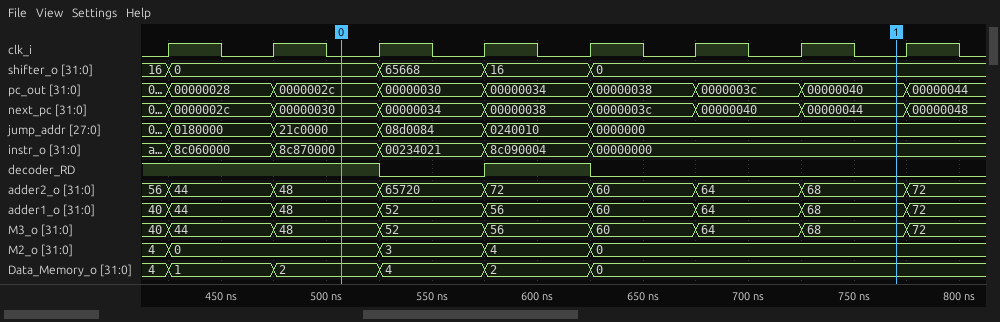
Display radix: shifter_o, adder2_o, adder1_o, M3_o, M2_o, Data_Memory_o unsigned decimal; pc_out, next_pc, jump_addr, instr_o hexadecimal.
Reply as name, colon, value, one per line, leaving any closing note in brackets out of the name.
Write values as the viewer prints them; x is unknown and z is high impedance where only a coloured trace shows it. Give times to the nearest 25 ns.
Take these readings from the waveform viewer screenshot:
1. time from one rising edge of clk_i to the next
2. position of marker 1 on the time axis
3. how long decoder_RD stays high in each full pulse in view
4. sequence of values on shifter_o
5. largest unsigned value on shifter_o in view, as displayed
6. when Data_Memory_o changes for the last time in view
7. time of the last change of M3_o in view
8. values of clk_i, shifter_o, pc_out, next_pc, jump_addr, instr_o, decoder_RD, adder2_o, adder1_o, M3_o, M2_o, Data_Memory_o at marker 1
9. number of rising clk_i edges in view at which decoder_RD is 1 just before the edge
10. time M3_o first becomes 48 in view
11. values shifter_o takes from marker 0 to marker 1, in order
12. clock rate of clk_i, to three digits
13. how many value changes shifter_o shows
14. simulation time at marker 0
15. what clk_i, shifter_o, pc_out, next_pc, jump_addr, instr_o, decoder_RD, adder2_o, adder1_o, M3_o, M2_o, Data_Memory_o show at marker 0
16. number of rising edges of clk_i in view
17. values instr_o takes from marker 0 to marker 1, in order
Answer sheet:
time from one rising edge of clk_i to the next: 50 ns
position of marker 1 on the time axis: 775 ns
how long decoder_RD stays high in each full pulse in view: 50 ns
sequence of values on shifter_o: 16, 0, 65668, 16, 0
largest unsigned value on shifter_o in view, as displayed: 65668
when Data_Memory_o changes for the last time in view: 625 ns
time of the last change of M3_o in view: 775 ns
values of clk_i, shifter_o, pc_out, next_pc, jump_addr, instr_o, decoder_RD, adder2_o, adder1_o, M3_o, M2_o, Data_Memory_o at marker 1: clk_i=0, shifter_o=0, pc_out=00000040, next_pc=00000044, jump_addr=0000000, instr_o=00000000, decoder_RD=0, adder2_o=68, adder1_o=68, M3_o=68, M2_o=0, Data_Memory_o=0
number of rising clk_i edges in view at which decoder_RD is 1 just before the edge: 4
time M3_o first becomes 48 in view: 475 ns
values shifter_o takes from marker 0 to marker 1, in order: 0, 65668, 16, 0
clock rate of clk_i, to three digits: 20.0 MHz
how many value changes shifter_o shows: 4
simulation time at marker 0: 500 ns
what clk_i, shifter_o, pc_out, next_pc, jump_addr, instr_o, decoder_RD, adder2_o, adder1_o, M3_o, M2_o, Data_Memory_o show at marker 0: clk_i=0, shifter_o=0, pc_out=0000002c, next_pc=00000030, jump_addr=21c0000, instr_o=8c870000, decoder_RD=1, adder2_o=48, adder1_o=48, M3_o=48, M2_o=0, Data_Memory_o=2
number of rising edges of clk_i in view: 8
values instr_o takes from marker 0 to marker 1, in order: 8c870000, 00234021, 8c090004, 00000000
